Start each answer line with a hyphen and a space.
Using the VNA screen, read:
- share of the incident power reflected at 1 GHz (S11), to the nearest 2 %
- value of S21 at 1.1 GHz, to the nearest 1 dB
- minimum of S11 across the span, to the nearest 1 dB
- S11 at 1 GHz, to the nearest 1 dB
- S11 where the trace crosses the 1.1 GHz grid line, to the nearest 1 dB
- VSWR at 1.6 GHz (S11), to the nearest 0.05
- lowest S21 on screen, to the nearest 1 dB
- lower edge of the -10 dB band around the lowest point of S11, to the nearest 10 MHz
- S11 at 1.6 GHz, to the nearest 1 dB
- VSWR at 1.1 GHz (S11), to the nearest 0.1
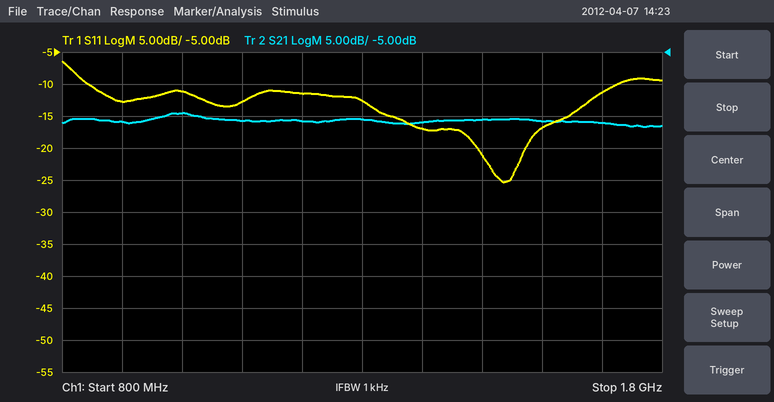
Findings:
- 8 %
- -16 dB
- -25 dB
- -11 dB
- -13 dB
- 1.35
- -17 dB
- 840 MHz
- -17 dB
- 1.6
